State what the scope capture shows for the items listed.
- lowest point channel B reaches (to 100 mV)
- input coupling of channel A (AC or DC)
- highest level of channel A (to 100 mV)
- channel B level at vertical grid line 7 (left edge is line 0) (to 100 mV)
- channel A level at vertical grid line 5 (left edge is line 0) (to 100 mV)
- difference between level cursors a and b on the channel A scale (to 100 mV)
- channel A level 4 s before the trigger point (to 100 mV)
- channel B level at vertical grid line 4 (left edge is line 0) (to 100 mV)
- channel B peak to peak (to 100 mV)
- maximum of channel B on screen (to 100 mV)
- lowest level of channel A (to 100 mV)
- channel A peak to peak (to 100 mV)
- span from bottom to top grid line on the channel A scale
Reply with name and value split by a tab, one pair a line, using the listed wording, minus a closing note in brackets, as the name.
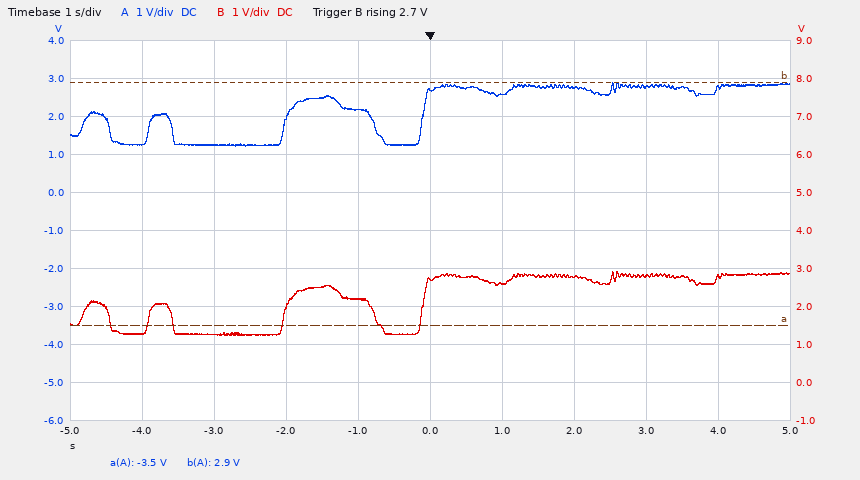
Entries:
lowest point channel B reaches	1.2 V
input coupling of channel A	DC
highest level of channel A	2.9 V
channel B level at vertical grid line 7 (left edge is line 0)	2.8 V
channel A level at vertical grid line 5 (left edge is line 0)	2.7 V
difference between level cursors a and b on the channel A scale	6.4 V
channel A level 4 s before the trigger point	1.3 V
channel B level at vertical grid line 4 (left edge is line 0)	2.2 V
channel B peak to peak	1.7 V
maximum of channel B on screen	2.9 V
lowest level of channel A	1.2 V
channel A peak to peak	1.7 V
span from bottom to top grid line on the channel A scale	10 V
